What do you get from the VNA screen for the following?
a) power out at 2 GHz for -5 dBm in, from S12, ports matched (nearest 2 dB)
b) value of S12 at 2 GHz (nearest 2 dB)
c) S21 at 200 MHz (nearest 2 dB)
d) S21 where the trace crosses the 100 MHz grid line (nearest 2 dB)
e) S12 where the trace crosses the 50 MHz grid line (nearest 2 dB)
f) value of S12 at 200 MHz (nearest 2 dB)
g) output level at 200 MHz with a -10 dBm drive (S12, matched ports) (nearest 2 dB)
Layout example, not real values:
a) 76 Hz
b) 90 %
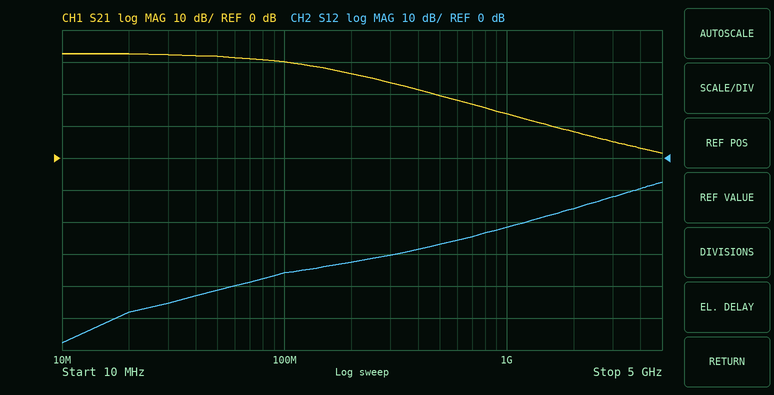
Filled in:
a) -20 dBm
b) -16 dB
c) 26 dB
d) 30 dB
e) -42 dB
f) -32 dB
g) -42 dBm
